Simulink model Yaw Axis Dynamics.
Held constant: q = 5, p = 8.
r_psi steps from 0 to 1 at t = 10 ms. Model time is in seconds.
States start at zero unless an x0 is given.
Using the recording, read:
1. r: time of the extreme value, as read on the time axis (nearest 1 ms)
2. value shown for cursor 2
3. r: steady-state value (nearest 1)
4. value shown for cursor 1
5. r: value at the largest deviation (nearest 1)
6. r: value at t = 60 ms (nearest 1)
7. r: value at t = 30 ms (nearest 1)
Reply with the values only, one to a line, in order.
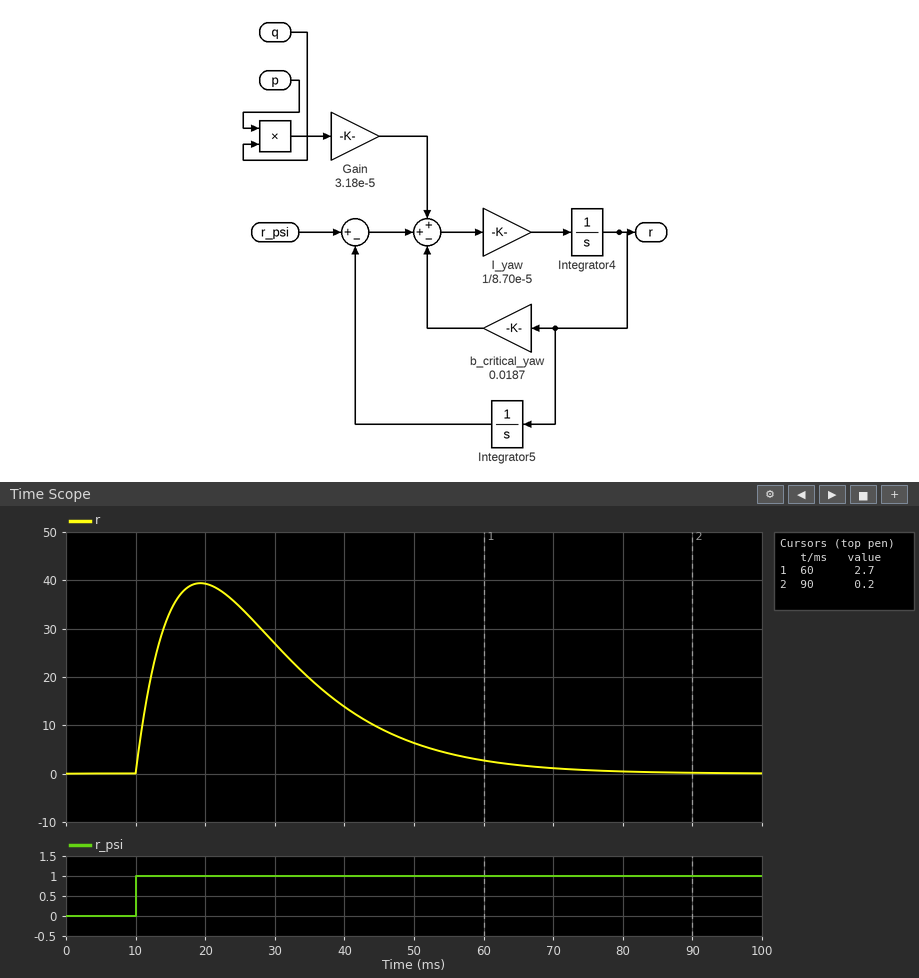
19 ms
0.2
0
2.7
39
3
27
